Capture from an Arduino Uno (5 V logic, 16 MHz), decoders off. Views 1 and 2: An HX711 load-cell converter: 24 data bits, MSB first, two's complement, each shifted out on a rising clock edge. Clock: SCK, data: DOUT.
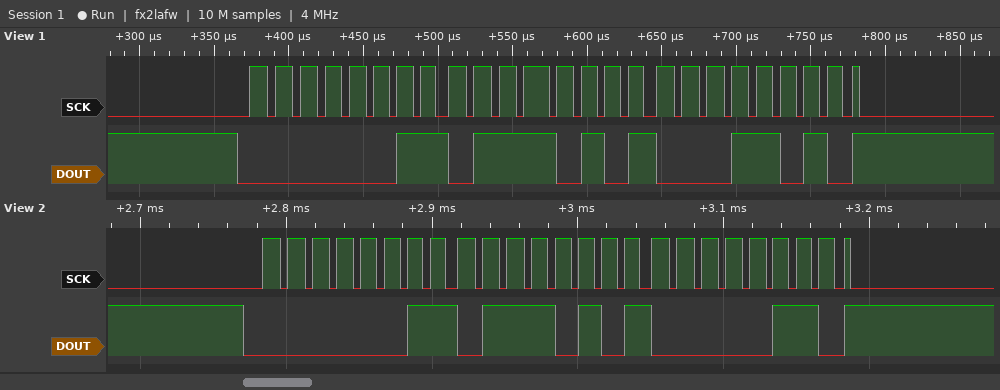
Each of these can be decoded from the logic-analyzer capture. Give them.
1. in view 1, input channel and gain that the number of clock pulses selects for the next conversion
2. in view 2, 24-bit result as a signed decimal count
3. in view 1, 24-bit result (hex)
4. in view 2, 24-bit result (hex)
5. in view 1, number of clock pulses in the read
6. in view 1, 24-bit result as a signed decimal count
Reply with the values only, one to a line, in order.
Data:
channel A, gain 128
226566
0x03751A
0x037506
25
226586
